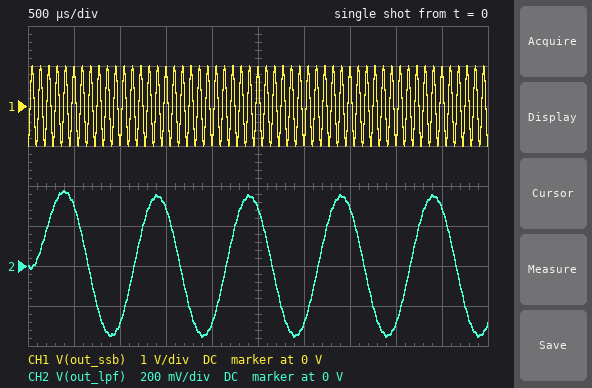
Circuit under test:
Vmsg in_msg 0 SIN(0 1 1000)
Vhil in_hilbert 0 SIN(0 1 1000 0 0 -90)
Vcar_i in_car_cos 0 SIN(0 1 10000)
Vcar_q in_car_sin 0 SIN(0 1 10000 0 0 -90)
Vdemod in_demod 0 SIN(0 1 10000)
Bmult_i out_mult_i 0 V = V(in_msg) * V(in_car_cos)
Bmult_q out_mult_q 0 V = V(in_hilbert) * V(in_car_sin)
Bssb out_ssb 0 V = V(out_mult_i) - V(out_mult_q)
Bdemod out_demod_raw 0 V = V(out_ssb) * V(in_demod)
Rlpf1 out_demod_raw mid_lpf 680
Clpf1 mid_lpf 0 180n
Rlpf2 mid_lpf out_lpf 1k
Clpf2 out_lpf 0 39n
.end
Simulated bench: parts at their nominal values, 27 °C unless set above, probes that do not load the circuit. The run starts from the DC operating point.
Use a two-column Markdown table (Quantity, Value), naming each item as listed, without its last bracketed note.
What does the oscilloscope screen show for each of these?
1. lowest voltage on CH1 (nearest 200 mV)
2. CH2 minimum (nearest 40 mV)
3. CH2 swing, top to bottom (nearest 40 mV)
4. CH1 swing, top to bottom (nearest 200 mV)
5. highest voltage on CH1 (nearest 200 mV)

| Quantity | Value |
|---|---|
| lowest voltage on CH1 | -1.0 V |
| CH2 minimum | -360 mV |
| CH2 swing, top to bottom | 720 mV |
| CH1 swing, top to bottom | 2.0 V |
| highest voltage on CH1 | 1.0 V |
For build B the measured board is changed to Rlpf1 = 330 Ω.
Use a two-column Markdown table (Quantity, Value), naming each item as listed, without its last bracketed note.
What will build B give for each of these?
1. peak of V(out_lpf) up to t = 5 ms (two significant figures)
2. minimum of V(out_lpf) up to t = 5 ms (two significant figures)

| Quantity | Value |
|---|---|
| peak of V(out_lpf) up to t = 5 ms | 450 mV |
| minimum of V(out_lpf) up to t = 5 ms | -450 mV |
